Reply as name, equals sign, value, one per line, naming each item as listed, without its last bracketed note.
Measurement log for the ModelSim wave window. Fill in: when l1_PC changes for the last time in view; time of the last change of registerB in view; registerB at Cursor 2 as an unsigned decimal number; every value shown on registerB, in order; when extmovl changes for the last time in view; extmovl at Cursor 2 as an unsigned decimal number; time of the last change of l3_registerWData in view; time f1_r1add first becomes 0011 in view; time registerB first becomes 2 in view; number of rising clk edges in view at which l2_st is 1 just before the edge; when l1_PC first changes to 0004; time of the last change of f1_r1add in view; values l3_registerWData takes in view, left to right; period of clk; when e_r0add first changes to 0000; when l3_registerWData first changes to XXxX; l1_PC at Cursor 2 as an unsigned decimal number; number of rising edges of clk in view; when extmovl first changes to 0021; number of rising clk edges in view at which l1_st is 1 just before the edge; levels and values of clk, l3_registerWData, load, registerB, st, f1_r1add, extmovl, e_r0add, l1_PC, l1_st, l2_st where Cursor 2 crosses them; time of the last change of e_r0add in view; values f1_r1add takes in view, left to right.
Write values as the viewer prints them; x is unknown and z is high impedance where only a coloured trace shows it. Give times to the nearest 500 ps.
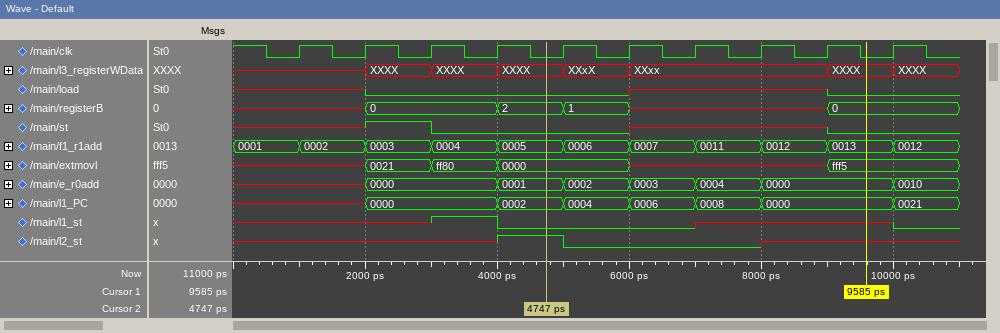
when l1_PC changes for the last time in view = 10000 ps
time of the last change of registerB in view = 9000 ps
registerB at Cursor 2 as an unsigned decimal number = 2
every value shown on registerB, in order = x, 0, 2, 1, x, 0
when extmovl changes for the last time in view = 9000 ps
extmovl at Cursor 2 as an unsigned decimal number = 0
time of the last change of l3_registerWData in view = 10000 ps
time f1_r1add first becomes 0011 in view = 7000 ps
time registerB first becomes 2 in view = 4000 ps
number of rising clk edges in view at which l2_st is 1 just before the edge = 1
when l1_PC first changes to 0004 = 5000 ps
time of the last change of f1_r1add in view = 10000 ps
values l3_registerWData takes in view, left to right = x, XXXX, XXXX, XXXX, XXxX, XXxx, XXXX, XXXX
period of clk = 1000 ps
when e_r0add first changes to 0000 = 2000 ps
when l3_registerWData first changes to XXxX = 5000 ps
l1_PC at Cursor 2 as an unsigned decimal number = 2
number of rising edges of clk in view = 10
when extmovl first changes to 0021 = 2000 ps
number of rising clk edges in view at which l1_st is 1 just before the edge = 1
levels and values of clk, l3_registerWData, load, registerB, st, f1_r1add, extmovl, e_r0add, l1_PC, l1_st, l2_st where Cursor 2 crosses them = clk=0, l3_registerWData=XXXX, load=0, registerB=2, st=0, f1_r1add=0005, extmovl=0000, e_r0add=0001, l1_PC=0002, l1_st=0, l2_st=1
time of the last change of e_r0add in view = 10000 ps
values f1_r1add takes in view, left to right = 0001, 0002, 0003, 0004, 0005, 0006, 0007, 0011, 0012, 0013, 0012
